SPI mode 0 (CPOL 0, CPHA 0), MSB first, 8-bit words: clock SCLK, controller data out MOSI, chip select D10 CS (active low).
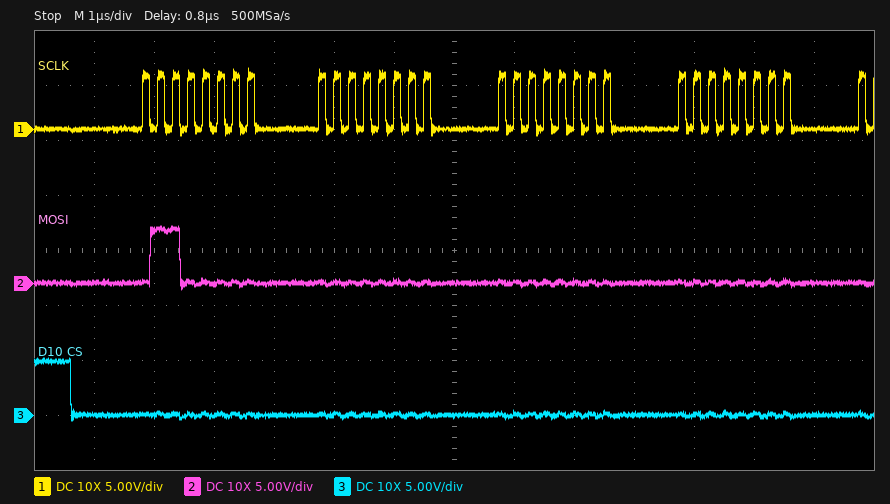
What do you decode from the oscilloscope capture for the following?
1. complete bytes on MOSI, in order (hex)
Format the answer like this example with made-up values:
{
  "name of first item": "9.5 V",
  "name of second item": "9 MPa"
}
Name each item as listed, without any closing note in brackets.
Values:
{
  "complete bytes on MOSI, in order": "60 00 00 00"
}
